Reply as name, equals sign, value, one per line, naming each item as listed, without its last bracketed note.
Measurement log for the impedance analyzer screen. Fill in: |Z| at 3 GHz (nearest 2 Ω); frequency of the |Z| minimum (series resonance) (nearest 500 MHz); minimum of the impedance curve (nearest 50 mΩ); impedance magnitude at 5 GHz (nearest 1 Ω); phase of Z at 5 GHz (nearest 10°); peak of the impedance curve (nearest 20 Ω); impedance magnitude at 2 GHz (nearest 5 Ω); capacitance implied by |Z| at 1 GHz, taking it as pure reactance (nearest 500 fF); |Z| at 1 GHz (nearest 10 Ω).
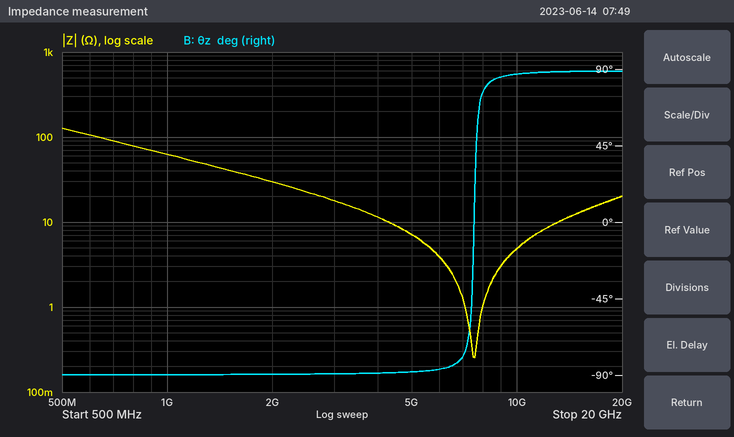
|Z| at 3 GHz = 18 Ω
frequency of the |Z| minimum (series resonance) = 7.5 GHz
minimum of the impedance curve = 250 mΩ
impedance magnitude at 5 GHz = 7 Ω
phase of Z at 5 GHz = -90°
peak of the impedance curve = 120 Ω
impedance magnitude at 2 GHz = 30 Ω
capacitance implied by |Z| at 1 GHz, taking it as pure reactance = 2.5 pF
|Z| at 1 GHz = 60 Ω
